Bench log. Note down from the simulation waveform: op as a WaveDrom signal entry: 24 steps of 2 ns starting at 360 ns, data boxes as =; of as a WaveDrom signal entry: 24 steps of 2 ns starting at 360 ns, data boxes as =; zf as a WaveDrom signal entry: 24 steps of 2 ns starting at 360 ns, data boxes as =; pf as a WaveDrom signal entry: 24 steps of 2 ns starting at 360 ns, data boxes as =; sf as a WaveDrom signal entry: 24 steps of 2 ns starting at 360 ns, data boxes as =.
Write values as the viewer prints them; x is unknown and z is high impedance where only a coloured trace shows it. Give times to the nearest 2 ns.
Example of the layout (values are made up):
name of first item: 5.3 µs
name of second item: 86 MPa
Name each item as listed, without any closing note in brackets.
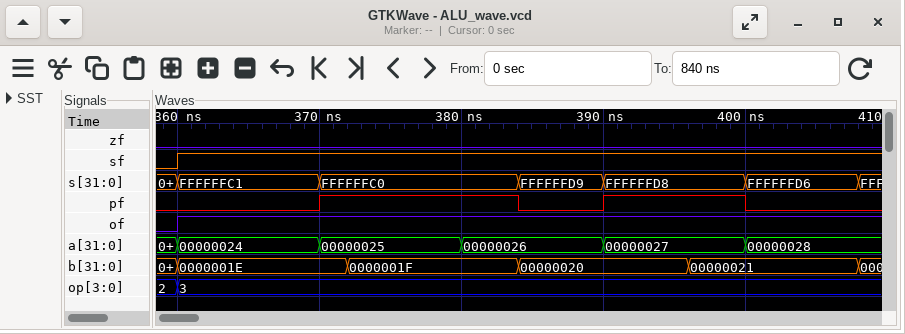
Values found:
op as a WaveDrom signal entry: 24 steps of 2 ns starting at 360 ns, data boxes as =: {name: 'op', wave: '=.......................', data: '3'}
of as a WaveDrom signal entry: 24 steps of 2 ns starting at 360 ns, data boxes as =: {name: 'of', wave: '1.......................'}
zf as a WaveDrom signal entry: 24 steps of 2 ns starting at 360 ns, data boxes as =: {name: 'zf', wave: '0.......................'}
pf as a WaveDrom signal entry: 24 steps of 2 ns starting at 360 ns, data boxes as =: {name: 'pf', wave: '0....1......0..1....0...'}
sf as a WaveDrom signal entry: 24 steps of 2 ns starting at 360 ns, data boxes as =: {name: 'sf', wave: '1.......................'}
